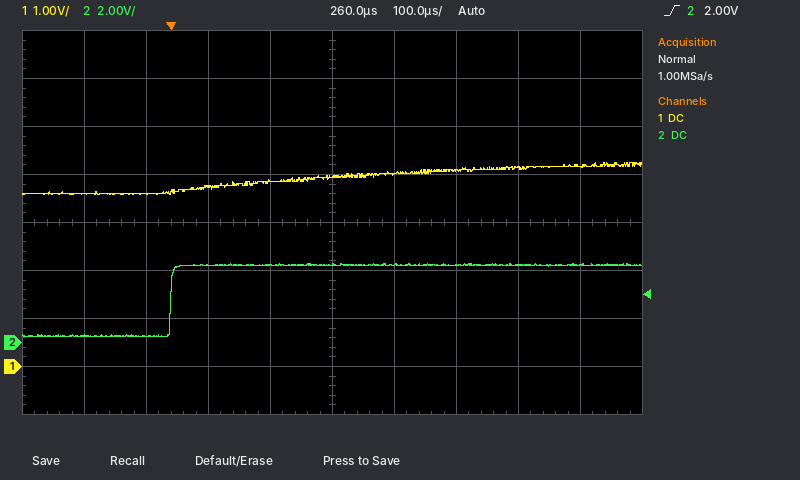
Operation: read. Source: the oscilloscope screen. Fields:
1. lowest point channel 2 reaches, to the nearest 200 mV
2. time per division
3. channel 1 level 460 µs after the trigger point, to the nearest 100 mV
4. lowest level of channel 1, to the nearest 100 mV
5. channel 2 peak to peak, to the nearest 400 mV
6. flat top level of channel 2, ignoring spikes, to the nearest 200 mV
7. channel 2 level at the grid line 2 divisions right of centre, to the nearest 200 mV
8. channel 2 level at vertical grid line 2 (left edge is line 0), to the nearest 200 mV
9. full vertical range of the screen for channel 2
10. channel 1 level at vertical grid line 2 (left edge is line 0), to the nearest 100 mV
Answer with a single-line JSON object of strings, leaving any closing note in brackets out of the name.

{"lowest point channel 2 reaches, to the nearest 200 mV": "200 mV", "time per division": "100 µs", "channel 1 level 460 µs after the trigger point, to the nearest 100 mV": "4.1 V", "lowest level of channel 1, to the nearest 100 mV": "3.6 V", "channel 2 peak to peak, to the nearest 400 mV": "3.2 V", "flat top level of channel 2, ignoring spikes, to the nearest 200 mV": "3.2 V", "channel 2 level at the grid line 2 divisions right of centre, to the nearest 200 mV": "3.2 V", "channel 2 level at vertical grid line 2 (left edge is line 0), to the nearest 200 mV": "200 mV", "full vertical range of the screen for channel 2": "16 V", "channel 1 level at vertical grid line 2 (left edge is line 0), to the nearest 100 mV": "3.6 V"}
